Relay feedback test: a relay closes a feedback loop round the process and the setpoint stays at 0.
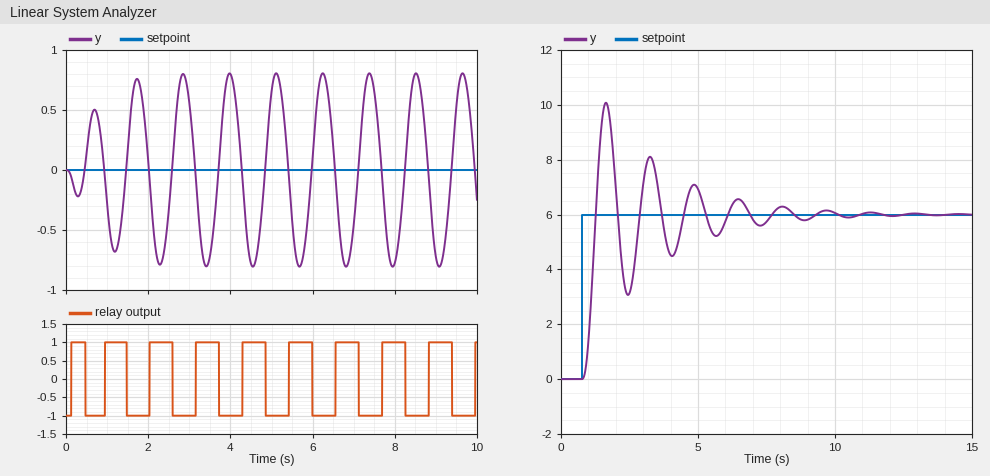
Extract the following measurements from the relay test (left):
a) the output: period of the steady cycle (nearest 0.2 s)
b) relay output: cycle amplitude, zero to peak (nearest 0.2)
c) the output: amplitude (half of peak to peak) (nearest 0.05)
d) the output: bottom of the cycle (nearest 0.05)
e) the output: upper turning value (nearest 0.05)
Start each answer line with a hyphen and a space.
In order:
- 1.2 s
- 1.0
- 0.80
- -0.80
- 0.80
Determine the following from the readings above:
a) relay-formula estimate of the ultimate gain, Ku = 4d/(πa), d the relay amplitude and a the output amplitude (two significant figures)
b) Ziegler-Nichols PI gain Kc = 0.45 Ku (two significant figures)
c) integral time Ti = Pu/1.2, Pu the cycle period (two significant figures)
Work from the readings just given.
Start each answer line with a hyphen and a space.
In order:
- 1.6
- 0.72
- 1.0 s
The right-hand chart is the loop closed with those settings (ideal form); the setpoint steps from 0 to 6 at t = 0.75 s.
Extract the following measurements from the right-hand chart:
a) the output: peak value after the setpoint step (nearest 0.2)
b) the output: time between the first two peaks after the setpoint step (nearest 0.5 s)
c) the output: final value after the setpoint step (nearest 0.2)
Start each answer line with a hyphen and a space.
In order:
- 10.0
- 1.5 s
- 6.0
